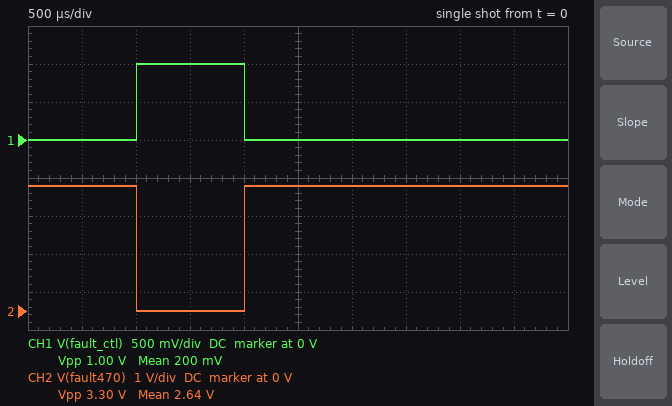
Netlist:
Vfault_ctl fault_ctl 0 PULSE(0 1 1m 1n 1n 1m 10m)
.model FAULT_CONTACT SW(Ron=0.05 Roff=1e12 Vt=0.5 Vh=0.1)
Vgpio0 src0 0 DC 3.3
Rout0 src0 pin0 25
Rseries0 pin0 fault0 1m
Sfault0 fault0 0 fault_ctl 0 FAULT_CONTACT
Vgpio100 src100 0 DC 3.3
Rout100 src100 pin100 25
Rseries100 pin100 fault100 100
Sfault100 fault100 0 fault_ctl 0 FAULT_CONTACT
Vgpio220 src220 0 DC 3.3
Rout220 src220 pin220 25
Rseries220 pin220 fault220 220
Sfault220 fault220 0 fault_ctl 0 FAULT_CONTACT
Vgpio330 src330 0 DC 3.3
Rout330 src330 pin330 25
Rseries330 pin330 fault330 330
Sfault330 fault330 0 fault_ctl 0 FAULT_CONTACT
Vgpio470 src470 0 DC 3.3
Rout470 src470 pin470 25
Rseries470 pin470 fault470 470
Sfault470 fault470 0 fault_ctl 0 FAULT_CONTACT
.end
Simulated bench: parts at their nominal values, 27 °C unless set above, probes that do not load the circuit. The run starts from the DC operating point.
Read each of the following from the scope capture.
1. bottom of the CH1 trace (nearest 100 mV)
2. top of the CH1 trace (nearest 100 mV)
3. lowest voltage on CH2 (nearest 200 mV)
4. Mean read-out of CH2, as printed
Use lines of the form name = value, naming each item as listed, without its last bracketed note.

bottom of the CH1 trace = 0 V
top of the CH1 trace = 1.0 V
lowest voltage on CH2 = 0 V
Mean read-out of CH2, as printed = 2.64 V
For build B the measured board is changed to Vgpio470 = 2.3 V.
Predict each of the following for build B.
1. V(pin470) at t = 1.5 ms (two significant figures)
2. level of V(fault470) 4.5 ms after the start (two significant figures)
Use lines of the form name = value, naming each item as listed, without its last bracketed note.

V(pin470) at t = 1.5 ms = 2.2 V
level of V(fault470) 4.5 ms after the start = 2.3 V
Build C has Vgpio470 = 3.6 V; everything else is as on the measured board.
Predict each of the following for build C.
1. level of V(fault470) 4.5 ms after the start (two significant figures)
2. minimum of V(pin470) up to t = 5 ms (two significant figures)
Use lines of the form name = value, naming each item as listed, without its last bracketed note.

level of V(fault470) 4.5 ms after the start = 3.6 V
minimum of V(pin470) up to t = 5 ms = 3.4 V
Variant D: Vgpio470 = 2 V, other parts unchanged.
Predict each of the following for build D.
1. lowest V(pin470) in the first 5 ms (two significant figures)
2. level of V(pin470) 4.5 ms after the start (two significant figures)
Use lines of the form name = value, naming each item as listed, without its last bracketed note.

lowest V(pin470) in the first 5 ms = 1.9 V
level of V(pin470) 4.5 ms after the start = 2.0 V
